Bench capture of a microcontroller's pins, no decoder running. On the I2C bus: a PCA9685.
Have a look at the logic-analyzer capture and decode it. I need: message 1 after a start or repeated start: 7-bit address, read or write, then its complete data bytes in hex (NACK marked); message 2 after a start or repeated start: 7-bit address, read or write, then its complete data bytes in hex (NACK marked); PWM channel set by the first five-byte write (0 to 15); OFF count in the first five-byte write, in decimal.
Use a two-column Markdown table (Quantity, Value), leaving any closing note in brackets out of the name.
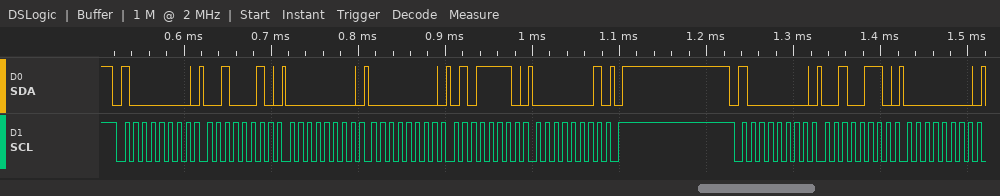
| Quantity | Value |
|---|---|
| message 1 after a start or repeated start: 7-bit address, read or write, then its complete data bytes in hex | 0x40 write: 22 00 00 5E 01 |
| message 2 after a start or repeated start: 7-bit address, read or write, then its complete data bytes in hex | 0x40 write: 26 00 |
| PWM channel set by the first five-byte write | 7 |
| OFF count in the first five-byte write, in decimal | 350 |
